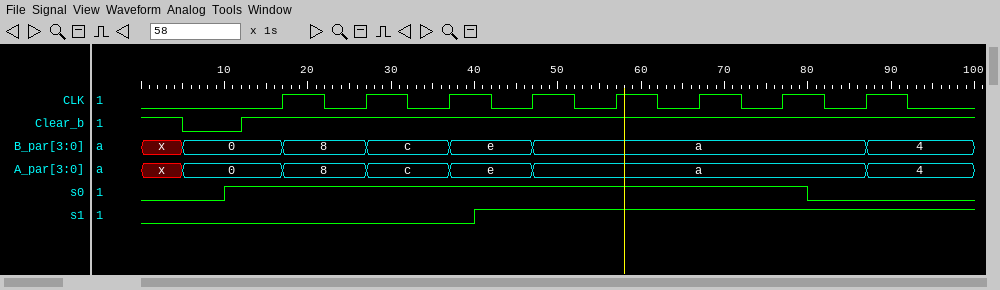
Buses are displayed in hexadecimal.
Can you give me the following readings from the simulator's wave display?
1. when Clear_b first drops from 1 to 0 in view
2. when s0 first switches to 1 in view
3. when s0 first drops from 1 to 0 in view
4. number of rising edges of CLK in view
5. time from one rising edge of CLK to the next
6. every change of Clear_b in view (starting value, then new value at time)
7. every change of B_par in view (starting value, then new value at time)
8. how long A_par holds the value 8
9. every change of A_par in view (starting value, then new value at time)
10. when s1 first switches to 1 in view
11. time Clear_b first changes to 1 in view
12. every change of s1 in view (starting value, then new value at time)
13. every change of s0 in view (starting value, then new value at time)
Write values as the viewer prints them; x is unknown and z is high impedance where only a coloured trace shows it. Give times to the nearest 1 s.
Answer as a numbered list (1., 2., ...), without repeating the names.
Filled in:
1. 5 s
2. 10 s
3. 80 s
4. 8
5. 10 s
6. 1, 0 at 5 s, 1 at 12 s
7. x, 0 at 5 s, 8 at 17 s, c at 27 s, e at 37 s, a at 47 s, 4 at 87 s
8. 10 s
9. x, 0 at 5 s, 8 at 17 s, c at 27 s, e at 37 s, a at 47 s, 4 at 87 s
10. 40 s
11. 12 s
12. 0, 1 at 40 s
13. 0, 1 at 10 s, 0 at 80 s
